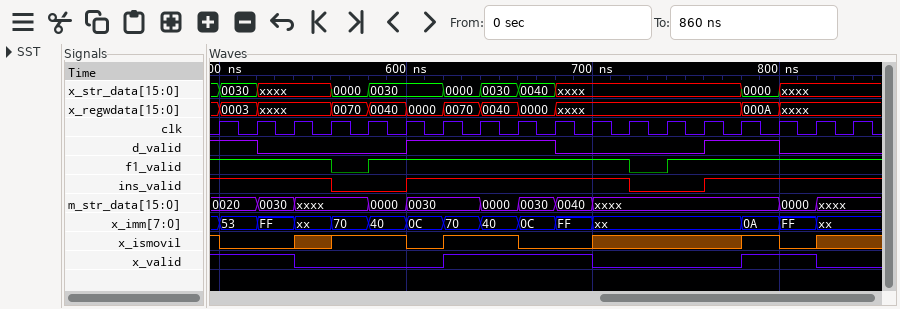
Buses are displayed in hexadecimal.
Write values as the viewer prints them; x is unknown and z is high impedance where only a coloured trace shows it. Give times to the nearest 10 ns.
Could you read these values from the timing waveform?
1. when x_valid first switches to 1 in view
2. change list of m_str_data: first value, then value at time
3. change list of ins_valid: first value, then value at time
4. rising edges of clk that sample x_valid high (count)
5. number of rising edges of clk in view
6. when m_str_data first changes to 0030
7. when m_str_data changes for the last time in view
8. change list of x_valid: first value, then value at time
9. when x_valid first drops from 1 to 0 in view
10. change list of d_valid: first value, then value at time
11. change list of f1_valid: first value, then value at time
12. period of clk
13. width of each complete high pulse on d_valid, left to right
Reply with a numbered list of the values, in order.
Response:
1. 620 ns
2. 0020, 0030 at 520 ns, xxxx at 540 ns, 0000 at 580 ns, 0030 at 600 ns, 0000 at 640 ns, 0030 at 660 ns, 0040 at 680 ns, xxxx at 700 ns, 0000 at 800 ns, xxxx at 820 ns
3. 1, 0 at 560 ns, 1 at 600 ns, 0 at 720 ns, 1 at 760 ns
4. 9
5. 18
6. 520 ns
7. 820 ns
8. 1, 0 at 540 ns, 1 at 620 ns, 0 at 700 ns, 1 at 780 ns, 0 at 820 ns
9. 540 ns
10. 1, 0 at 520 ns, 1 at 600 ns, 0 at 680 ns, 1 at 760 ns, 0 at 800 ns
11. 1, 0 at 560 ns, 1 at 580 ns, 0 at 720 ns, 1 at 740 ns
12. 20 ns
13. 80 ns, 40 ns
